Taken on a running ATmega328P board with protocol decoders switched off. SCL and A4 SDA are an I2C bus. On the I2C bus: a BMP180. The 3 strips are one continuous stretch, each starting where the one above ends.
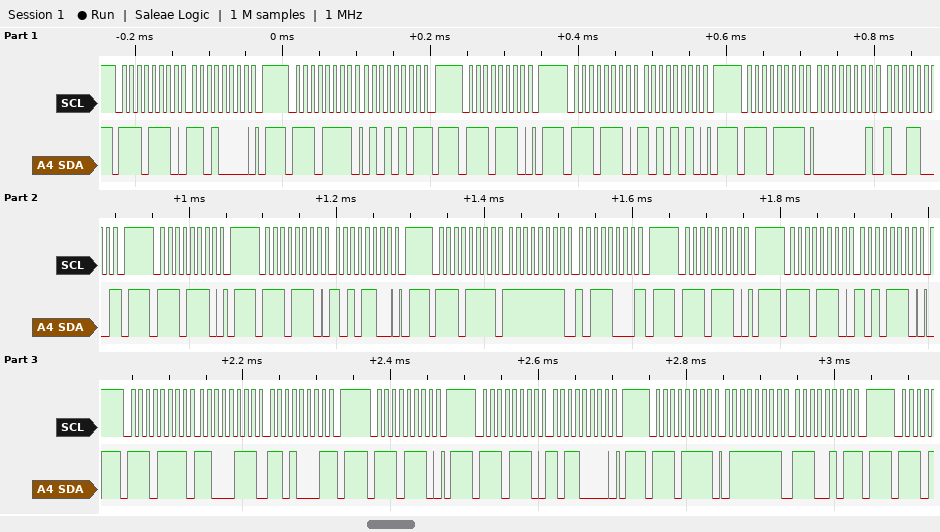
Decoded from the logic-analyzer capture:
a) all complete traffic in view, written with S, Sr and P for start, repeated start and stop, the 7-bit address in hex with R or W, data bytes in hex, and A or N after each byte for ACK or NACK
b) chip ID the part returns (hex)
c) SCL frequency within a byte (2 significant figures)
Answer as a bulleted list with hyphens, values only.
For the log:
- S 77W A D0 A P S 77R A 55 N P S 77W A P S 77W A AA A P S 77R A 01 A 98 N P S 77W A P S 77W A AC A P S 77R A FF A B8 N P S 77W A P S 77W A AE A P S 77R A C7 A D1 N P S 77W A P S 77W A B0 A P S 77R A 7F A E5 N P
- 0x55
- 100 kHz
